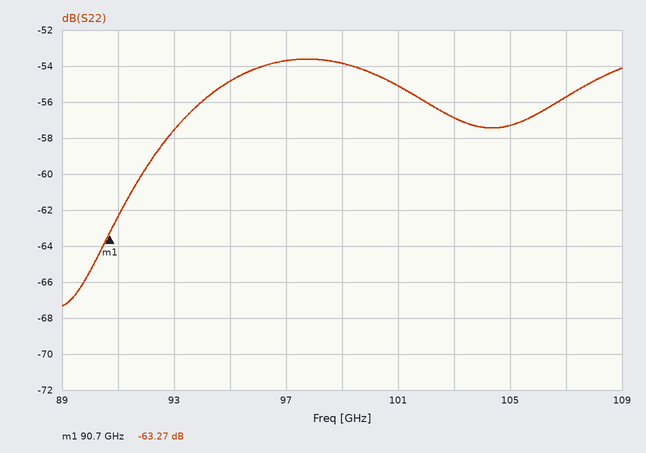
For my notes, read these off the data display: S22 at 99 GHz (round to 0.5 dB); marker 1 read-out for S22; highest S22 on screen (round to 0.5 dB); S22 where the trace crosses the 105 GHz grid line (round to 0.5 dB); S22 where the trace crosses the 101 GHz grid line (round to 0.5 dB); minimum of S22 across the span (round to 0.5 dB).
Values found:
-54.0 dB
-63.27 dB
-53.5 dB
-57.5 dB
-55.0 dB
-67.5 dB
